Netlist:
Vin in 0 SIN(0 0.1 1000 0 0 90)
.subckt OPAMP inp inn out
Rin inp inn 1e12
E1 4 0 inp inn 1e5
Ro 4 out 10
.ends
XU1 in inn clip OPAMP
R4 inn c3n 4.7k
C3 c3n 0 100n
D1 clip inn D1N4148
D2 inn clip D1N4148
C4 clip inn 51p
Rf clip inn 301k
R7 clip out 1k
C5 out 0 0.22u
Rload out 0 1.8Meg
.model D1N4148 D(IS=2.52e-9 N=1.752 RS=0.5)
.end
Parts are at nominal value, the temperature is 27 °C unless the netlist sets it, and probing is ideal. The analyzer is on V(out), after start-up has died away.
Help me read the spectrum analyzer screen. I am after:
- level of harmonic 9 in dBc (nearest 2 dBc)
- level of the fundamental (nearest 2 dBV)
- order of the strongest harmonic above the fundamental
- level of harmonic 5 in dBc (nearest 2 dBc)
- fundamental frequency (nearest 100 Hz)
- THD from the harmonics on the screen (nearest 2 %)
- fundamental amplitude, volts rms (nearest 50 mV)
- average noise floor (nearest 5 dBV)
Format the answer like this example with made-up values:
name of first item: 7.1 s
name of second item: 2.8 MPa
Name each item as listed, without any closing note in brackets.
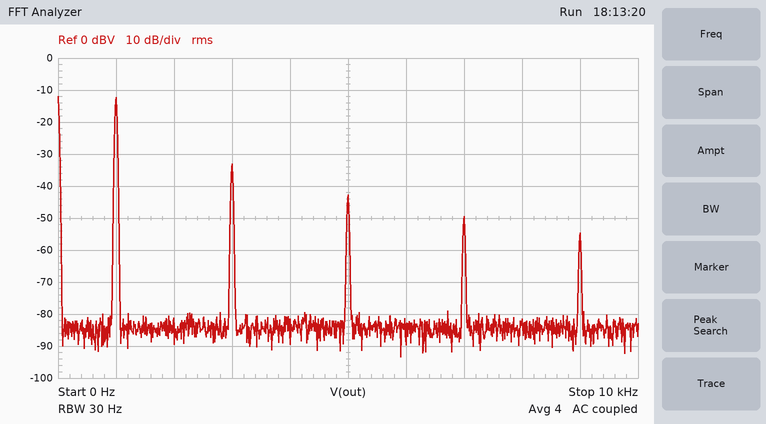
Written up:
level of harmonic 9 in dBc: -42 dBc
level of the fundamental: -12 dBV
order of the strongest harmonic above the fundamental: 3
level of harmonic 5 in dBc: -30 dBc
fundamental frequency: 1.0 kHz
THD from the harmonics on the screen: 10 %
fundamental amplitude, volts rms: 250 mV
average noise floor: -85 dBV
